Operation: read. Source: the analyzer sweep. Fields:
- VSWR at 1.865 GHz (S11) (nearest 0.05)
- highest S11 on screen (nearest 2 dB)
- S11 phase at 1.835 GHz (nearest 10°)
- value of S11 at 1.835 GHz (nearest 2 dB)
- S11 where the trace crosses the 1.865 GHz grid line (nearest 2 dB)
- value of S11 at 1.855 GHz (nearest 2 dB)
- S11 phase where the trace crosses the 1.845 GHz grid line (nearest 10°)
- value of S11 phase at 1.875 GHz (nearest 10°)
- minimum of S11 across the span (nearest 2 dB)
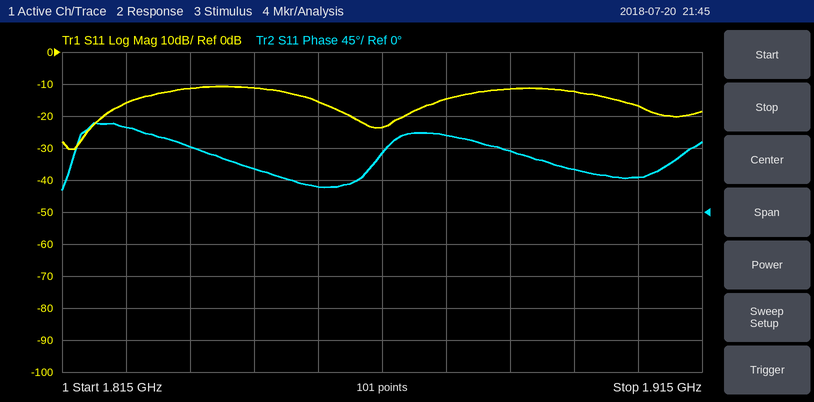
1.15
-10 dB
90°
-12 dB
-24 dB
-16 dB
60°
110°
-30 dB
